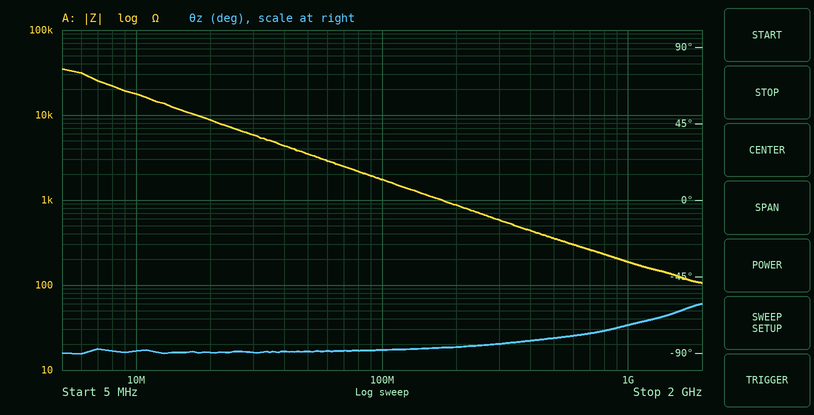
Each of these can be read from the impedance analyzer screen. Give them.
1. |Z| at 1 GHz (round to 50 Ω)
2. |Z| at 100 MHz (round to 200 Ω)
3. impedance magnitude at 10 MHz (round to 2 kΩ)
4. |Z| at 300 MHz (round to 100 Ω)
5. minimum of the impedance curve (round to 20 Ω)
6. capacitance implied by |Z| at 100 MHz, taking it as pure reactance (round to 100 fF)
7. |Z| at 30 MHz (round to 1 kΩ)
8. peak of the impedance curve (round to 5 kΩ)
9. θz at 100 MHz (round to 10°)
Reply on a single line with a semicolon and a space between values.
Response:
200 Ω; 1.8 kΩ; 18 kΩ; 600 Ω; 100 Ω; 900 fF; 6 kΩ; 35 kΩ; -90°
